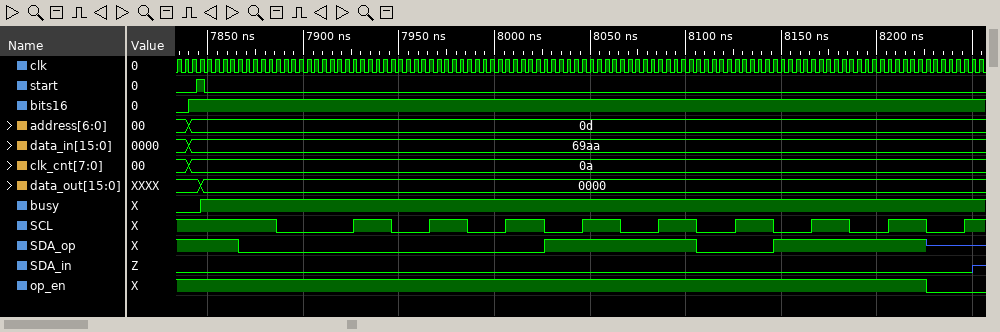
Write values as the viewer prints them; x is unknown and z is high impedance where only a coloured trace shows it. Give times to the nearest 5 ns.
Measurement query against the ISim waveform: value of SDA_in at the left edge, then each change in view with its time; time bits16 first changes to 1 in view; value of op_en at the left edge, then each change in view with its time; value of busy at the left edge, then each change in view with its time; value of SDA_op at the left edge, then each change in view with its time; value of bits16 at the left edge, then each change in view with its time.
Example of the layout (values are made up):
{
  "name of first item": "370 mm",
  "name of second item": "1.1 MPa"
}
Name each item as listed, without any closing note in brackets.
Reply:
{
  "value of SDA_in at the left edge, then each change in view with its time": "0, z at 8250 ns",
  "time bits16 first changes to 1 in view": "7840 ns",
  "value of op_en at the left edge, then each change in view with its time": "1, 0 at 8225 ns",
  "value of busy at the left edge, then each change in view with its time": "0, 1 at 7845 ns",
  "value of SDA_op at the left edge, then each change in view with its time": "1, 0 at 7865 ns, 1 at 8025 ns, 0 at 8105 ns, 1 at 8145 ns, z at 8225 ns",
  "value of bits16 at the left edge, then each change in view with its time": "0, 1 at 7840 ns"
}
